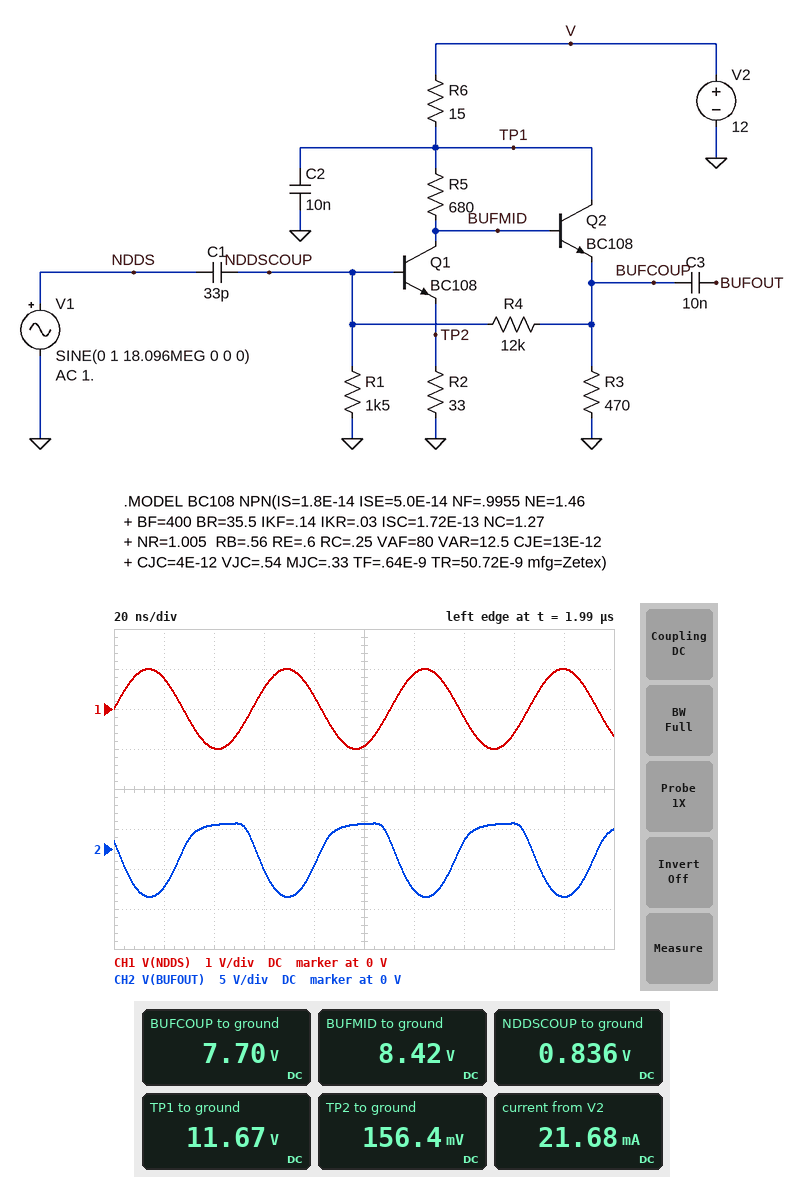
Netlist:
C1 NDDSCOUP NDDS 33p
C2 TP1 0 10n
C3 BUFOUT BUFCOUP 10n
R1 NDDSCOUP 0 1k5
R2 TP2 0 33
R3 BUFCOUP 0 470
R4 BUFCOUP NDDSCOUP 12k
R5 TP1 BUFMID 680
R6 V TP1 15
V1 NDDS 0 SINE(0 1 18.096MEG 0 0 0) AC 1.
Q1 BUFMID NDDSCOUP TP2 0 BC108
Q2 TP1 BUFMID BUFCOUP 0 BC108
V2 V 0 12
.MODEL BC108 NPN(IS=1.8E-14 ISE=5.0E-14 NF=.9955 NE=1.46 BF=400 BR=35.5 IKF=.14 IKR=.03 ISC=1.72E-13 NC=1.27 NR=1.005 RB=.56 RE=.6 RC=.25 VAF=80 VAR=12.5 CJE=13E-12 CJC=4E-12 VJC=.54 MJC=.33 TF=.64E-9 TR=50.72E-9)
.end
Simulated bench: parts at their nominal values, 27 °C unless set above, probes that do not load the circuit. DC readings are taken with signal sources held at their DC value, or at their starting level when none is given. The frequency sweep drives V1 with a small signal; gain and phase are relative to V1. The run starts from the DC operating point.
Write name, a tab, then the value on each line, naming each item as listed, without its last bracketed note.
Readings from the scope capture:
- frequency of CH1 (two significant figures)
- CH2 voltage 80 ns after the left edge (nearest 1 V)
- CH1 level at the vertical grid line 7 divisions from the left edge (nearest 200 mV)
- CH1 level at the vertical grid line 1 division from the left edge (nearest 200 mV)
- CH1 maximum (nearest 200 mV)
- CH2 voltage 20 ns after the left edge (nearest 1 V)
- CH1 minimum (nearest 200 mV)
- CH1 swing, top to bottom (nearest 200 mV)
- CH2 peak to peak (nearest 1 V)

frequency of CH1	18 MHz
CH2 voltage 80 ns after the left edge	-2 V
CH1 level at the vertical grid line 7 divisions from the left edge	-200 mV
CH1 level at the vertical grid line 1 division from the left edge	800 mV
CH1 maximum	1.0 V
CH2 voltage 20 ns after the left edge	-5 V
CH1 minimum	-1.0 V
CH1 swing, top to bottom	2.0 V
CH2 peak to peak	9 V
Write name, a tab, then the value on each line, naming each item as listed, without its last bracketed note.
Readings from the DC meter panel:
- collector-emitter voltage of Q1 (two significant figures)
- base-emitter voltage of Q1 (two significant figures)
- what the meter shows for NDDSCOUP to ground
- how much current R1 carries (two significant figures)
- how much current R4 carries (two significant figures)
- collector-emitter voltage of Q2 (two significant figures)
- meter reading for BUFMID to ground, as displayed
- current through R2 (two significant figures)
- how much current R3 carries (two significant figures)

collector-emitter voltage of Q1	8.3 V
base-emitter voltage of Q1	680 mV
what the meter shows for NDDSCOUP to ground	0.836 V
how much current R1 carries	560 µA
how much current R4 carries	570 µA
collector-emitter voltage of Q2	4.0 V
meter reading for BUFMID to ground, as displayed	8.42 V
current through R2	4.7 mA
how much current R3 carries	16 mA
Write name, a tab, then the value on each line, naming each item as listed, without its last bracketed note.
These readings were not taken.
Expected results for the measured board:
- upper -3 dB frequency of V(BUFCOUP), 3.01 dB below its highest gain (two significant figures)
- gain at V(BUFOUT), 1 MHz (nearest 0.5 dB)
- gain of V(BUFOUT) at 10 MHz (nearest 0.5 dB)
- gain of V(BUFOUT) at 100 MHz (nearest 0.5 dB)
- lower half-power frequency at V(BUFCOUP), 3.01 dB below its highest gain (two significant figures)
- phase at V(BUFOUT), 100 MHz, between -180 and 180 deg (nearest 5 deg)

upper -3 dB frequency of V(BUFCOUP), 3.01 dB below its highest gain	75 MHz
gain at V(BUFOUT), 1 MHz	3.5 dB
gain of V(BUFOUT) at 10 MHz	16.0 dB
gain of V(BUFOUT) at 100 MHz	12.0 dB
lower half-power frequency at V(BUFCOUP), 3.01 dB below its highest gain	4.0 MHz
phase at V(BUFOUT), 100 MHz, between -180 and 180 deg	115 deg
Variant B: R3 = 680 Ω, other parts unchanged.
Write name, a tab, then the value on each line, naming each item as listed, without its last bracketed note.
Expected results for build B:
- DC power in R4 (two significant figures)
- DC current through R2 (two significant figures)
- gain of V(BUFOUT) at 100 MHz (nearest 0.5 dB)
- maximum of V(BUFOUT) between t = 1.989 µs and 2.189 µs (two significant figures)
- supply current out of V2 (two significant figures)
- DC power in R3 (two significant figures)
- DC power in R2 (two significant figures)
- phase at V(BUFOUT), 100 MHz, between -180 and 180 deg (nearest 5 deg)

DC power in R4	4.0 mW
DC current through R2	4.8 mA
gain of V(BUFOUT) at 100 MHz	12.5 dB
maximum of V(BUFOUT) between t = 1.989 µs and 2.189 µs	3.3 V
supply current out of V2	17 mA
DC power in R3	88 mW
DC power in R2	770 µW
phase at V(BUFOUT), 100 MHz, between -180 and 180 deg	115 deg
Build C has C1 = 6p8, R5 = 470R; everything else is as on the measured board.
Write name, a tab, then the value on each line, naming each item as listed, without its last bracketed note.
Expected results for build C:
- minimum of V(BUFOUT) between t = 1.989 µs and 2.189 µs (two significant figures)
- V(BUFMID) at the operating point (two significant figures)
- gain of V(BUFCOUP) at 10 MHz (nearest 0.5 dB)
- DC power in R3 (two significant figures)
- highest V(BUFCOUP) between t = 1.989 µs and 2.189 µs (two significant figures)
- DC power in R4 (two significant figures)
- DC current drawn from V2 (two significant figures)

minimum of V(BUFOUT) between t = 1.989 µs and 2.189 µs	-1.6 V
V(BUFMID) at the operating point	8.9 V
gain of V(BUFCOUP) at 10 MHz	3.5 dB
DC power in R3	140 mW
highest V(BUFCOUP) between t = 1.989 µs and 2.189 µs	9.7 V
DC power in R4	4.4 mW
DC current drawn from V2	24 mA
